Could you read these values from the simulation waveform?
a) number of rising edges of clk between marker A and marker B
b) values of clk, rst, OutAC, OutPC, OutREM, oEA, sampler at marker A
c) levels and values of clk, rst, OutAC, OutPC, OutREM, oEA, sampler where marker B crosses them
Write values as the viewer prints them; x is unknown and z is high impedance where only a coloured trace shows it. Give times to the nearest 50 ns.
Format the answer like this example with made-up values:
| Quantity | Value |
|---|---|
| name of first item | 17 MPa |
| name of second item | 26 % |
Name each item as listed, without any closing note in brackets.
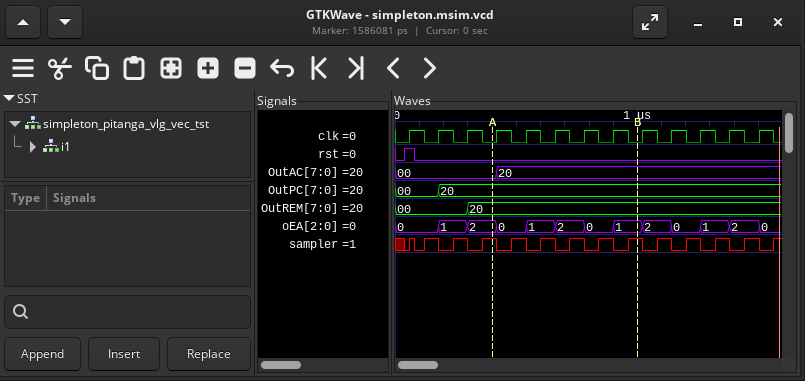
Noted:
| Quantity | Value |
|---|---|
| number of rising edges of clk between marker A and marker B | 5 |
| values of clk, rst, OutAC, OutPC, OutREM, oEA, sampler at marker A | clk=0, rst=0, OutAC=00, OutPC=20, OutREM=20, oEA=2, sampler=1 |
| levels and values of clk, rst, OutAC, OutPC, OutREM, oEA, sampler where marker B crosses them | clk=0, rst=0, OutAC=20, OutPC=20, OutREM=20, oEA=1, sampler=1 |
